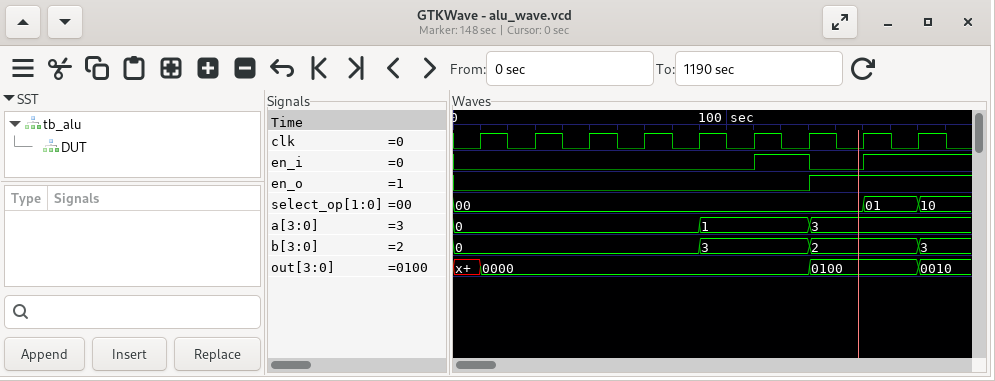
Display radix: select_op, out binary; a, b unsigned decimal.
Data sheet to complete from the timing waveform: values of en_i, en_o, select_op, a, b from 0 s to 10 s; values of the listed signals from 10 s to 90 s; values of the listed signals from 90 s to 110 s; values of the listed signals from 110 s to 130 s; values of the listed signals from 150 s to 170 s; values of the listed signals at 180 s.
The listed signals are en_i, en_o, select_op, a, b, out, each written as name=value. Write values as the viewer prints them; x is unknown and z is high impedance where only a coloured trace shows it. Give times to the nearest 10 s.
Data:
en_i=0, en_o=0, select_op=00, a=0, b=0
en_i=0, en_o=0, select_op=00, a=0, b=0, out=0000
en_i=0, en_o=0, select_op=00, a=1, b=3, out=0000
en_i=1, en_o=0, select_op=00, a=1, b=3, out=0000
en_i=1, en_o=1, select_op=01, a=3, b=2, out=0100
en_i=1, en_o=1, select_op=10, a=3, b=3, out=0010
